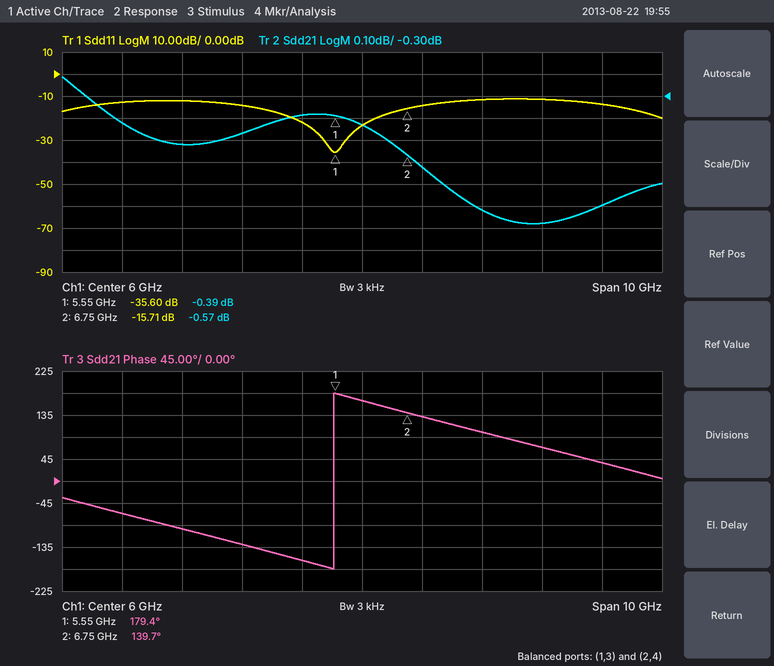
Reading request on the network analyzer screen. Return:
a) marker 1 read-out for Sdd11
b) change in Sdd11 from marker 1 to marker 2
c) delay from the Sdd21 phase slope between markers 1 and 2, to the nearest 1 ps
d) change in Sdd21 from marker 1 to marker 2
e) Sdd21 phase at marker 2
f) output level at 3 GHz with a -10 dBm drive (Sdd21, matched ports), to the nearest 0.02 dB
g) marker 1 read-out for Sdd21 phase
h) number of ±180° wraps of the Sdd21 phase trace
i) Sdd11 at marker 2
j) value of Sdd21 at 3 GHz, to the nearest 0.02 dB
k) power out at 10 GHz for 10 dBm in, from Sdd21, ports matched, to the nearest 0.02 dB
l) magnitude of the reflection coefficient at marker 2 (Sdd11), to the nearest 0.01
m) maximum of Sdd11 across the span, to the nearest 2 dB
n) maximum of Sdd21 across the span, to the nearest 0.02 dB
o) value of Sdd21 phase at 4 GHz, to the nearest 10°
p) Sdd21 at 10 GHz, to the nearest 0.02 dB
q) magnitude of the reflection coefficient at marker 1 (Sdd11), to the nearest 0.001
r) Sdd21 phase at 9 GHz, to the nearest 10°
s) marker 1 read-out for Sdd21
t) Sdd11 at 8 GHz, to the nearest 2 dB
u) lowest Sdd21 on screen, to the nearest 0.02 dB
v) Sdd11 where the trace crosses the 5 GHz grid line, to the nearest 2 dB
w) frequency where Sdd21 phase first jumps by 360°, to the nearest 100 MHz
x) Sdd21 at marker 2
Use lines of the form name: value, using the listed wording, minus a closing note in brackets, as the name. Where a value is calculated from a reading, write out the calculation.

marker 1 read-out for Sdd11: -35.60 dB
change in Sdd11 from marker 1 to marker 2: -15.71 − (-35.6) = 19.89 dB
delay from the Sdd21 phase slope between markers 1 and 2, to the nearest 1 ps: −(139.7° − (179.4°))/(360° × 1.2 GHz) ≈ 92 ps
change in Sdd21 from marker 1 to marker 2: -0.57 − (-0.39) = -0.18 dB
Sdd21 phase at marker 2: 139.7°
output level at 3 GHz with a -10 dBm drive (Sdd21, matched ports), to the nearest 0.02 dB: -10 dBm + (-0.52 dB) = -10.52 dBm
marker 1 read-out for Sdd21 phase: 179.4°
number of ±180° wraps of the Sdd21 phase trace: 1
Sdd11 at marker 2: -15.71 dB
value of Sdd21 at 3 GHz, to the nearest 0.02 dB: -0.52 dB
power out at 10 GHz for 10 dBm in, from Sdd21, ports matched, to the nearest 0.02 dB: 10 dBm + (-0.80 dB) = 9.20 dBm
magnitude of the reflection coefficient at marker 2 (Sdd11), to the nearest 0.01: 10^(-15.71/20) ≈ 0.16
maximum of Sdd11 across the span, to the nearest 2 dB: -12 dB
maximum of Sdd21 across the span, to the nearest 0.02 dB: -0.22 dB
value of Sdd21 phase at 4 GHz, to the nearest 10°: -130°
Sdd21 at 10 GHz, to the nearest 0.02 dB: -0.80 dB
magnitude of the reflection coefficient at marker 1 (Sdd11), to the nearest 0.001: 10^(-35.6/20) ≈ 0.017
Sdd21 phase at 9 GHz, to the nearest 10°: 70°
marker 1 read-out for Sdd21: -0.39 dB
Sdd11 at 8 GHz, to the nearest 2 dB: -12 dB
lowest Sdd21 on screen, to the nearest 0.02 dB: -0.88 dB
Sdd11 where the trace crosses the 5 GHz grid line, to the nearest 2 dB: -22 dB
frequency where Sdd21 phase first jumps by 360°, to the nearest 100 MHz: 5.5 GHz
Sdd21 at marker 2: -0.57 dB
